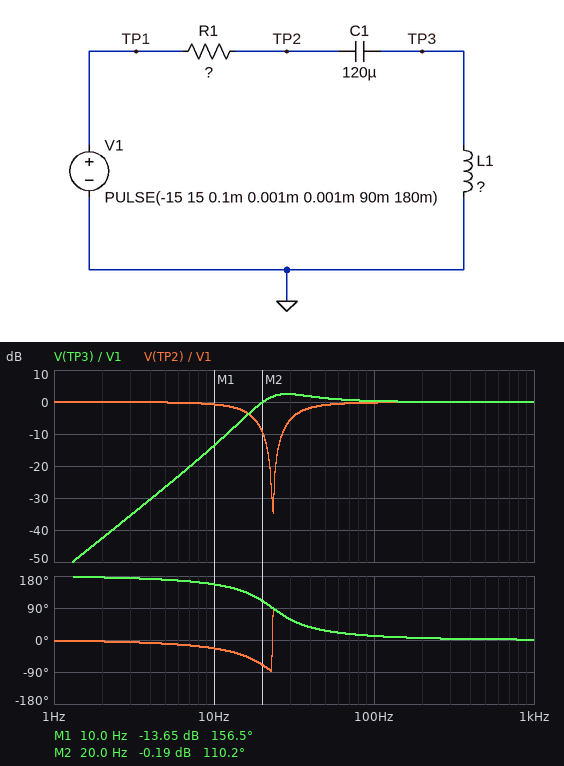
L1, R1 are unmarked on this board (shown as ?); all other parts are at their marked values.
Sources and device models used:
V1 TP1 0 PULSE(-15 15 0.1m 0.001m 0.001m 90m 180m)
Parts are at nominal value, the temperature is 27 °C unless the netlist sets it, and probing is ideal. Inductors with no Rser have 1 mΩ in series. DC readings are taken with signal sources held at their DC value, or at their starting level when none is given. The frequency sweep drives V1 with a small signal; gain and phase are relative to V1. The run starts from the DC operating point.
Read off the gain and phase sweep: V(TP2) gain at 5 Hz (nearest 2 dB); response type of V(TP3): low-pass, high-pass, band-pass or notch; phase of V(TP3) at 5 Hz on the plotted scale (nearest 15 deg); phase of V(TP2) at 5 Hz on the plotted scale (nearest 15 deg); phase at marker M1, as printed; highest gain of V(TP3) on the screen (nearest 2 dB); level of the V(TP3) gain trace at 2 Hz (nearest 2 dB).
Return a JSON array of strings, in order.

["0 dB", "high-pass", "165 deg", "-15 deg", "156.5 deg", "2 dB", "-42 dB"]
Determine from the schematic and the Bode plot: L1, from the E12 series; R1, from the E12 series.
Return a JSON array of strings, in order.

["390 mH", "47 Ω"]
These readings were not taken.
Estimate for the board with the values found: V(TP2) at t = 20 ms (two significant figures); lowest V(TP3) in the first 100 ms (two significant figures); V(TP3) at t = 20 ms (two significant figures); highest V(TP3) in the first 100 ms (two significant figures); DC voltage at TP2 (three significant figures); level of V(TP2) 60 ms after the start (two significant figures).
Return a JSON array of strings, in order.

["11 V", "-30 V", "-9.9 V", "30 V", "-15.0 V", "14 V"]
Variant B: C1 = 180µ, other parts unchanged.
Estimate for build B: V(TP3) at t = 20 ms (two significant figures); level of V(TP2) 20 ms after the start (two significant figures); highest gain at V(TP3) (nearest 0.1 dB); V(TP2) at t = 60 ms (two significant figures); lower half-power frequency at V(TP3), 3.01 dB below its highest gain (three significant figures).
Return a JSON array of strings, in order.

["-8.9 V", "5.6 V", "1.2 dB", "15 V", "16.3 Hz"]
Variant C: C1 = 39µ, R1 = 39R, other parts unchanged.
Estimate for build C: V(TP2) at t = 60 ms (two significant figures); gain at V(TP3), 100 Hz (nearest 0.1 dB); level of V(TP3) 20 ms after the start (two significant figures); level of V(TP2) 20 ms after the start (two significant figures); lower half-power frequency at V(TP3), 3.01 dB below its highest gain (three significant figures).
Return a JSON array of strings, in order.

["15 V", "1.4 dB", "5.3 V", "19 V", "35.7 Hz"]
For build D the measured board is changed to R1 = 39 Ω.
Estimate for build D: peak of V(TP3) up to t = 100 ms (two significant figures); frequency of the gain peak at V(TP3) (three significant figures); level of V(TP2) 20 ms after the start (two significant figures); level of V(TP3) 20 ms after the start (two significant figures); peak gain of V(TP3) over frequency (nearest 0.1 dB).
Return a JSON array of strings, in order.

["30 V", "26.6 Hz", "12 V", "-12 V", "3.8 dB"]
